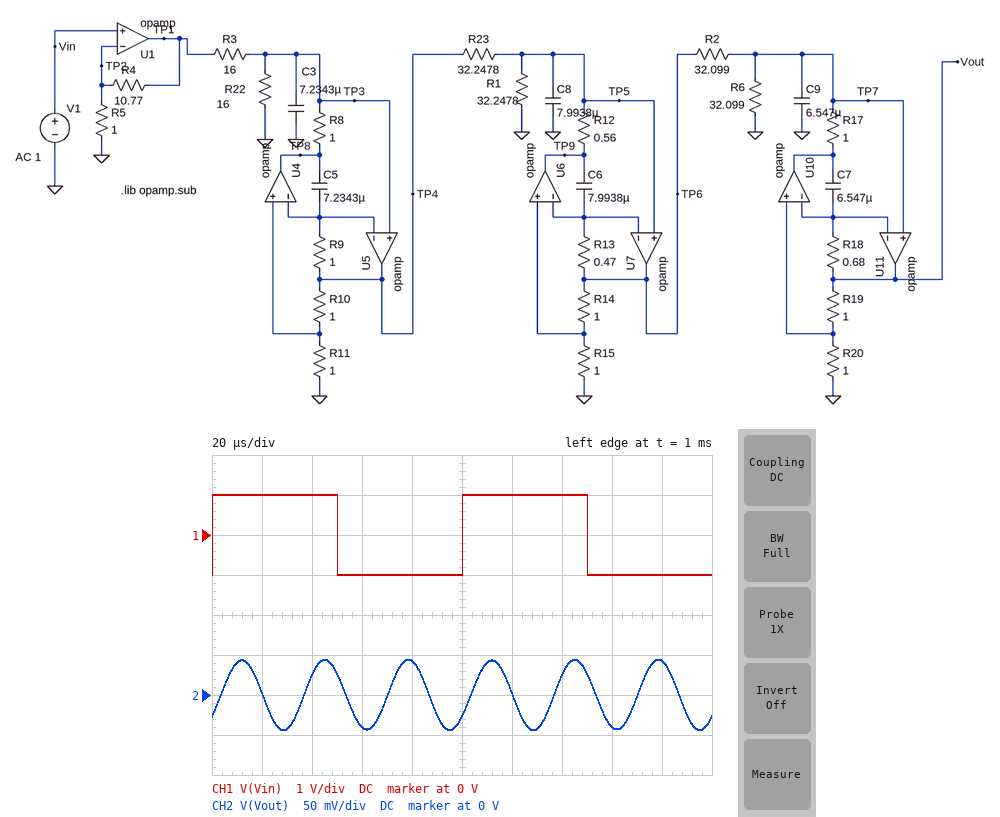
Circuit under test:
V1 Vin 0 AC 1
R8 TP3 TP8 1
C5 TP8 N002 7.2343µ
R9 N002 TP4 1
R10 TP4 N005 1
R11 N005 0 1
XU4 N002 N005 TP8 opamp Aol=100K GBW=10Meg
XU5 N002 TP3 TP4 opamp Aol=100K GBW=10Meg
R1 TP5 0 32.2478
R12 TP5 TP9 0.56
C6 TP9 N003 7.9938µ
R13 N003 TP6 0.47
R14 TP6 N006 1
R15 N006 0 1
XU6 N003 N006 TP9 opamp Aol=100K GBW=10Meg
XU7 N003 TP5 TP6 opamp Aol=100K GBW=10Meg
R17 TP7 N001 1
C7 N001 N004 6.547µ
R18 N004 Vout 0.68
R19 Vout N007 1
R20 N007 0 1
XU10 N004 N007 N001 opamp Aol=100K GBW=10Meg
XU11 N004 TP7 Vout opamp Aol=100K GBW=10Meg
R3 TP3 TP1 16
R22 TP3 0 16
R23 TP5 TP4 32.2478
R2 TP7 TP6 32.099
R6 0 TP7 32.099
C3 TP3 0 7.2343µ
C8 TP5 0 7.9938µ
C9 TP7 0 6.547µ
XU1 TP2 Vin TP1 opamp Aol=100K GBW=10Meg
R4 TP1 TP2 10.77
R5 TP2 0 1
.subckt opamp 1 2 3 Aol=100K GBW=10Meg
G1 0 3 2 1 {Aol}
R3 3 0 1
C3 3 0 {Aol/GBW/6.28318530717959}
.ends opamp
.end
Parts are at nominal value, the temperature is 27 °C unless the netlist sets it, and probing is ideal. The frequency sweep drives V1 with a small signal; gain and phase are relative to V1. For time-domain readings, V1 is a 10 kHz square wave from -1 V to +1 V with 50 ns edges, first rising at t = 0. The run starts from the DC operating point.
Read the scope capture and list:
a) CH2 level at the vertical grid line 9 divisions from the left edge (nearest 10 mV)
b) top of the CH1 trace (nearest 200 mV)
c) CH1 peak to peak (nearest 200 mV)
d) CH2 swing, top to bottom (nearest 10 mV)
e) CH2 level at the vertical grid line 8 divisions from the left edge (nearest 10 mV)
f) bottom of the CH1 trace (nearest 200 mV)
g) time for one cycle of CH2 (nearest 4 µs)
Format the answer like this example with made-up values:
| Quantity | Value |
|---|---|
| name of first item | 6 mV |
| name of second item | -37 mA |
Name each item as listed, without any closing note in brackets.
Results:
| Quantity | Value |
|---|---|
| CH2 level at the vertical grid line 9 divisions from the left edge | 40 mV |
| top of the CH1 trace | 1.0 V |
| CH1 peak to peak | 2.0 V |
| CH2 swing, top to bottom | 90 mV |
| CH2 level at the vertical grid line 8 divisions from the left edge | -40 mV |
| bottom of the CH1 trace | -1.0 V |
| time for one cycle of CH2 | 32 µs |
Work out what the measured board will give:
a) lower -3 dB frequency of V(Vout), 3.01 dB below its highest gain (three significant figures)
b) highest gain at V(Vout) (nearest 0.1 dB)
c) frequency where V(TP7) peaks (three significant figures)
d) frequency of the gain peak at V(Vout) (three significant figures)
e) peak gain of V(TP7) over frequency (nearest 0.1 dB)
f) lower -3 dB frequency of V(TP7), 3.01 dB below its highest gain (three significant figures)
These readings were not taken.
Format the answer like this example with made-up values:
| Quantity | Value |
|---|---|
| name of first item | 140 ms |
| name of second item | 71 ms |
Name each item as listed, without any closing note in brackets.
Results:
| Quantity | Value |
|---|---|
| lower -3 dB frequency of V(Vout), 3.01 dB below its highest gain | 28.6 kHz |
| highest gain at V(Vout) | -17.2 dB |
| frequency where V(TP7) peaks | 29.3 kHz |
| frequency of the gain peak at V(Vout) | 29.3 kHz |
| peak gain of V(TP7) over frequency | -23.2 dB |
| lower -3 dB frequency of V(TP7), 3.01 dB below its highest gain | 28.6 kHz |
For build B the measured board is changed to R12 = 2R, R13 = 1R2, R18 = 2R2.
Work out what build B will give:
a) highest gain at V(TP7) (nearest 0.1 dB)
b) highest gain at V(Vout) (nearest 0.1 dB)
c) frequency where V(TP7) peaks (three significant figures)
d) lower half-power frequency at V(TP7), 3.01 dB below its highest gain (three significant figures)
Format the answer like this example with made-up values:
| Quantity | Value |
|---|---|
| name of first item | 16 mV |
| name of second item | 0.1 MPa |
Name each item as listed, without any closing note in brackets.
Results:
| Quantity | Value |
|---|---|
| highest gain at V(TP7) | -12.7 dB |
| highest gain at V(Vout) | -6.7 dB |
| frequency where V(TP7) peaks | 16.3 kHz |
| lower half-power frequency at V(TP7), 3.01 dB below its highest gain | 15.5 kHz |
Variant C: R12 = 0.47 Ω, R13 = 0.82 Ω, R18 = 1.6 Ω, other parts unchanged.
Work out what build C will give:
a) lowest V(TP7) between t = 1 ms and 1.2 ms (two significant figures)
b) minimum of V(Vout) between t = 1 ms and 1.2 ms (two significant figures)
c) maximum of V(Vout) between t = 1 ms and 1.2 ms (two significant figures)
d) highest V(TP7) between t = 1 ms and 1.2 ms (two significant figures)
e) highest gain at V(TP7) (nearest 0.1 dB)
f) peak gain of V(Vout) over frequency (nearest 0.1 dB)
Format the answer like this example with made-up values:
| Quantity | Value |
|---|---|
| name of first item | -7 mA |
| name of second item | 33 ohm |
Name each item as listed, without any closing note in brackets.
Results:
| Quantity | Value |
|---|---|
| lowest V(TP7) between t = 1 ms and 1.2 ms | -12 mV |
| minimum of V(Vout) between t = 1 ms and 1.2 ms | -25 mV |
| maximum of V(Vout) between t = 1 ms and 1.2 ms | 25 mV |
| highest V(TP7) between t = 1 ms and 1.2 ms | 12 mV |
| highest gain at V(TP7) | -20.5 dB |
| peak gain of V(Vout) over frequency | -14.5 dB |
